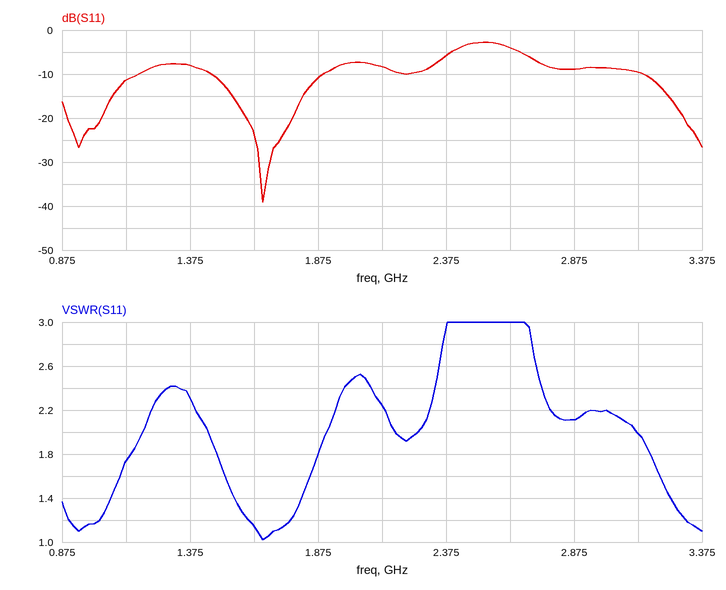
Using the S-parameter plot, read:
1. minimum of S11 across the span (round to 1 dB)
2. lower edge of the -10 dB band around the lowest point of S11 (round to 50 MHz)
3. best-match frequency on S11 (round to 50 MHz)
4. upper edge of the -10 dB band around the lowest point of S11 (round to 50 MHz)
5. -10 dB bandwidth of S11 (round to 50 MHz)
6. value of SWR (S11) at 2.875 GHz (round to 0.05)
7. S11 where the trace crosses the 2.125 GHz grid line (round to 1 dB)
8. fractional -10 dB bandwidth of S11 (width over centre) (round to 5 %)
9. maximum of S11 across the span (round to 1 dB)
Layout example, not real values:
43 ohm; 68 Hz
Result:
-39 dB; 1.45 GHz; 1.65 GHz; 1.90 GHz; 450 MHz; 2.10; -8 dB; 25 %; -3 dB
